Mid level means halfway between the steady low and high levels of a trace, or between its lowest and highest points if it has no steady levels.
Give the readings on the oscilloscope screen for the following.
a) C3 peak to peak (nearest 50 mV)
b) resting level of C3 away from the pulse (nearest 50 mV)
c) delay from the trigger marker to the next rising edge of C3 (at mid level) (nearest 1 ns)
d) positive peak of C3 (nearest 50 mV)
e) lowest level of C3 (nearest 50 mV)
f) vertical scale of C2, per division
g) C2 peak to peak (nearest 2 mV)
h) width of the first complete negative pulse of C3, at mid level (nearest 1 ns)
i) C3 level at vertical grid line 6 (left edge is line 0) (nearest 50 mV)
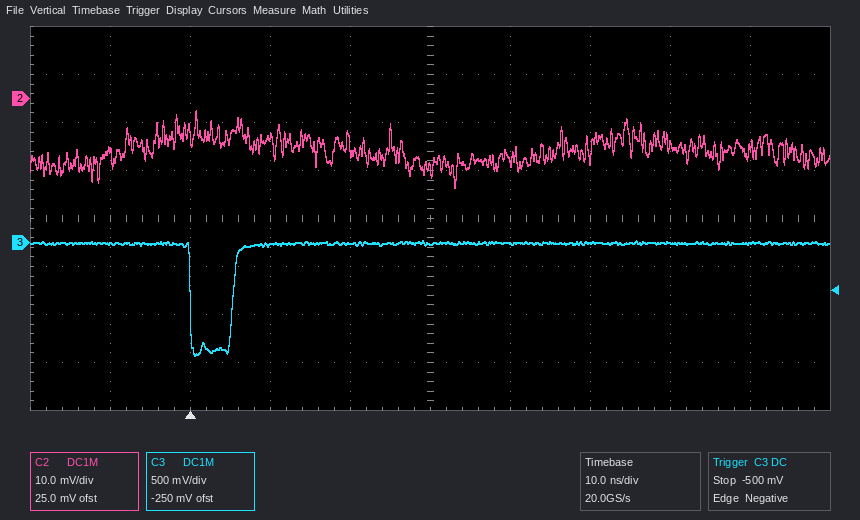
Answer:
1.20 V
0 mV
5 ns
0 mV
-1.20 V
10 mV
16 mV
5 ns
0 mV
